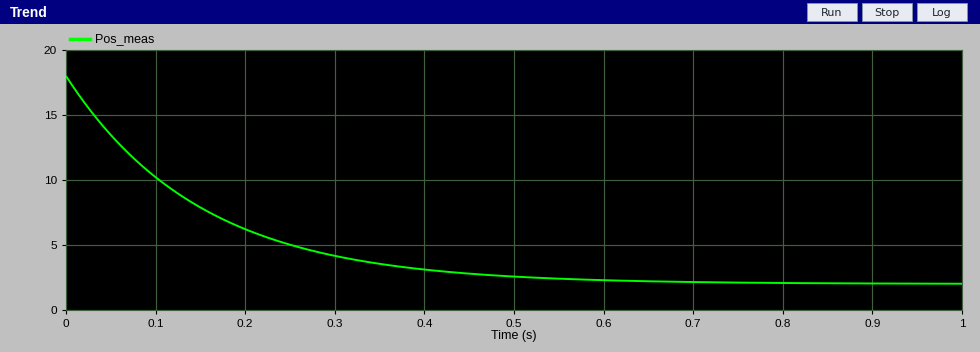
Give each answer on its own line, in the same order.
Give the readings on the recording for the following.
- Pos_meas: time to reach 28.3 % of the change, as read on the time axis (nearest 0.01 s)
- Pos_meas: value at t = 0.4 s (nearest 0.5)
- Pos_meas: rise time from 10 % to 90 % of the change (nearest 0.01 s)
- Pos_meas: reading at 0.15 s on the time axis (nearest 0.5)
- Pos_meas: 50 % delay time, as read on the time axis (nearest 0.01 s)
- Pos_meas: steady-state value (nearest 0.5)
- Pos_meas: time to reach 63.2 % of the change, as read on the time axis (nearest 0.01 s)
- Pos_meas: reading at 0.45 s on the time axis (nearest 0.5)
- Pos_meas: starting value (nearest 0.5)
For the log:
0.05 s
3.0
0.33 s
8.0
0.10 s
2.0
0.15 s
3.0
18.0
